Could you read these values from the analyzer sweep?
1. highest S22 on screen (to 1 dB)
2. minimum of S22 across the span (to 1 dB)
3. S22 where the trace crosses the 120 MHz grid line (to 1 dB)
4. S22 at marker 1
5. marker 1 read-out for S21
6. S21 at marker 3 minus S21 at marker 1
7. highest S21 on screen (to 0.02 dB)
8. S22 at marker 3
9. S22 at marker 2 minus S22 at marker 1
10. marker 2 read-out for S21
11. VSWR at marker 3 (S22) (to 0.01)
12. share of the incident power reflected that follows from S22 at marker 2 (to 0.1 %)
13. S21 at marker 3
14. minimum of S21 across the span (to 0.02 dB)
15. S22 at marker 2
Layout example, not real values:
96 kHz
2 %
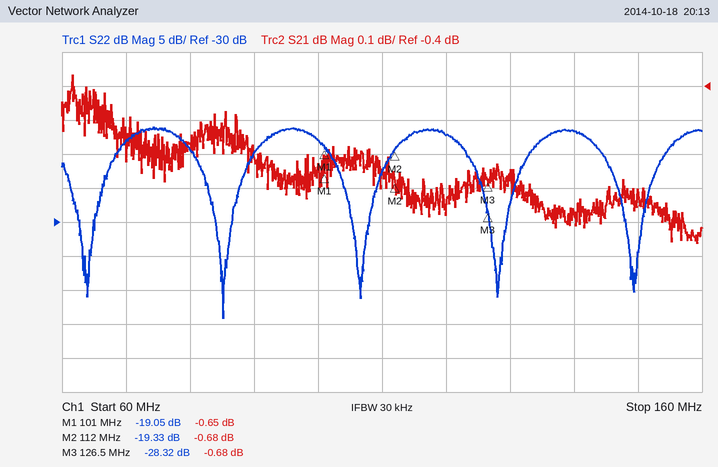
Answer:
-16 dB
-44 dB
-17 dB
-19.05 dB
-0.65 dB
-0.03 dB
-0.36 dB
-28.32 dB
-0.28 dB
-0.68 dB
1.08
1.2 %
-0.68 dB
-0.86 dB
-19.33 dB
